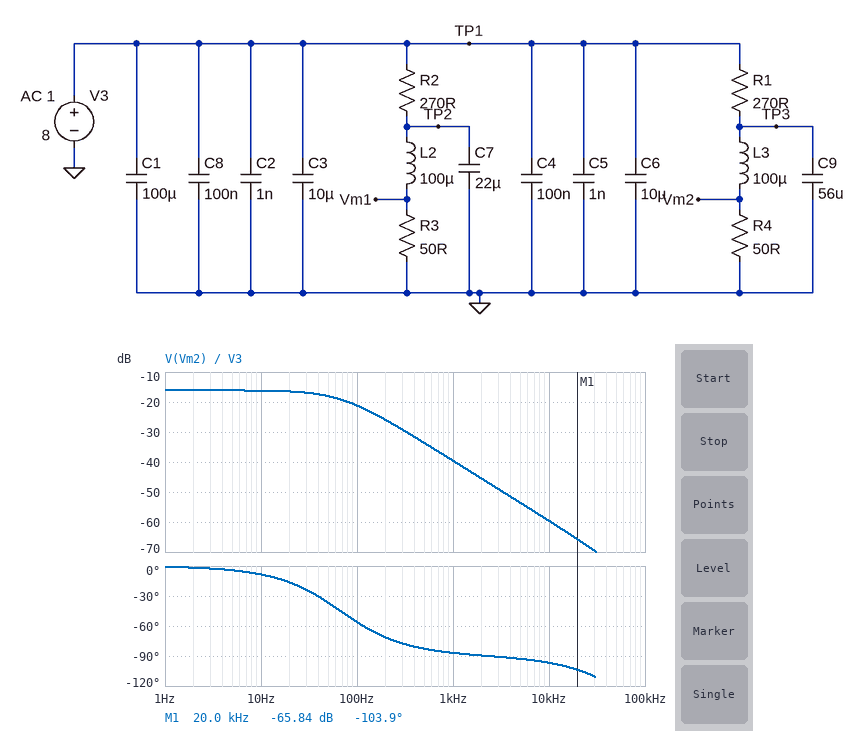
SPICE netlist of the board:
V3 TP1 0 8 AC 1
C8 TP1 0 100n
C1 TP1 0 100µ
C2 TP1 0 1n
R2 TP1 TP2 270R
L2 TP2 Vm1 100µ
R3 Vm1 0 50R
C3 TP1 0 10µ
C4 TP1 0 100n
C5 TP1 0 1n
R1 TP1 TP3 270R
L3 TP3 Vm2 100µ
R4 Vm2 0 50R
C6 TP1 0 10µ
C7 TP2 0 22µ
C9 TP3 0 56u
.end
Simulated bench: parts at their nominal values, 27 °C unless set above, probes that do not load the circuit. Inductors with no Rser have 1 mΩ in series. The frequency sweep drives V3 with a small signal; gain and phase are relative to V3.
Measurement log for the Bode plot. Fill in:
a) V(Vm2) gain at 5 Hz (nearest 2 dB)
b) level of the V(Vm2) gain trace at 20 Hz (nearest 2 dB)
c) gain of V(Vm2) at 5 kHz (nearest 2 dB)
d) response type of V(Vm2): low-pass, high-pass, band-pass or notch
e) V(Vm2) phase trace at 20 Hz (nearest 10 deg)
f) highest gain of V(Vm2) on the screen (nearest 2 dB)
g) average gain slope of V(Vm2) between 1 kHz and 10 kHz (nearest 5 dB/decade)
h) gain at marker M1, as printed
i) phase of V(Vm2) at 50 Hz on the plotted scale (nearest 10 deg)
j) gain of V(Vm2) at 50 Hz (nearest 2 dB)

-16 dB
-16 dB
-54 dB
low-pass
-20 deg
-16 dB
-20 dB/decade
-65.84 dB
-40 deg
-18 dB
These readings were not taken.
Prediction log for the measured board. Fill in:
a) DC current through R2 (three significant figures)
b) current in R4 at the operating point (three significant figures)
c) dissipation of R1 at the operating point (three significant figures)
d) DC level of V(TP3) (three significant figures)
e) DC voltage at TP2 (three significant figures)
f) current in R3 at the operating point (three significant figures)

25.0 mA
25.0 mA
169 mW
1.25 V
1.25 V
25.0 mA
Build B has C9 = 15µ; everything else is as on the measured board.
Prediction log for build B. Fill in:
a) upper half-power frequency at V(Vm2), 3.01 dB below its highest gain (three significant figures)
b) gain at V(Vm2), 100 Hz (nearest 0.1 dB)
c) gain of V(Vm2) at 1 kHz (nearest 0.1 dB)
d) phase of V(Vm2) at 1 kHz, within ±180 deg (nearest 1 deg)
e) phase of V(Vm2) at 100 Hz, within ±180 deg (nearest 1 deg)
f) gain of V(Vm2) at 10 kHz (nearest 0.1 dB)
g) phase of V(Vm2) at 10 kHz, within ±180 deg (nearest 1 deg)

252 Hz
-16.8 dB
-28.4 dB
-77 deg
-22 deg
-48.2 dB
-96 deg
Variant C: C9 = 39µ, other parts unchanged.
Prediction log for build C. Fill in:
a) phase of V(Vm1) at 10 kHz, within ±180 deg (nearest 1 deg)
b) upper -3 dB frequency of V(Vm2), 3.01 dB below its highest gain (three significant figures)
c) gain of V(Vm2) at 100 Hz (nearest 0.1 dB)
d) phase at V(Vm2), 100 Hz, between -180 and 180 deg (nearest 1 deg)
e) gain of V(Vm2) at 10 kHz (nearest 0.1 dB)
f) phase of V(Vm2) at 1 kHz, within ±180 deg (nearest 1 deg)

-96 deg
96.8 Hz
-19.3 dB
-46 deg
-56.5 dB
-85 deg
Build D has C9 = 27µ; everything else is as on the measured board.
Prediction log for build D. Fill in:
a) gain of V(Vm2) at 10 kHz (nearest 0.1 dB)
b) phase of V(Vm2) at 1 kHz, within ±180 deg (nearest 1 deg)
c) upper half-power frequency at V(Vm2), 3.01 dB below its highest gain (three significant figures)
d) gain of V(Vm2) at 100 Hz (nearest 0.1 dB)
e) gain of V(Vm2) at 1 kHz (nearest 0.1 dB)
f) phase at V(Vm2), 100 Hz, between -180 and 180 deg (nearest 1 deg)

-53.3 dB
-83 deg
140 Hz
-17.9 dB
-33.3 dB
-36 deg
